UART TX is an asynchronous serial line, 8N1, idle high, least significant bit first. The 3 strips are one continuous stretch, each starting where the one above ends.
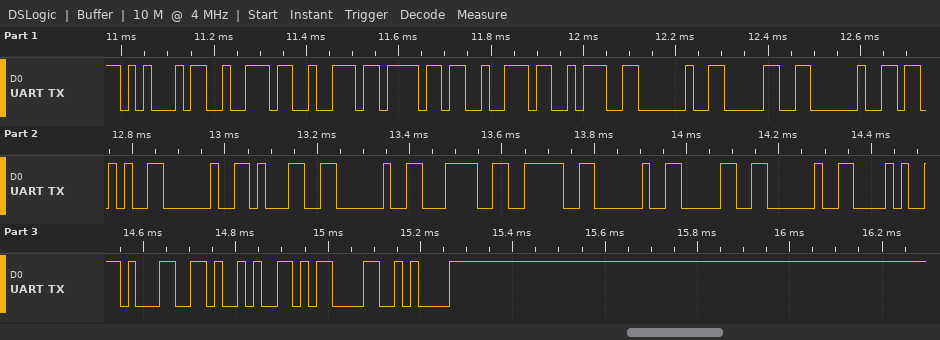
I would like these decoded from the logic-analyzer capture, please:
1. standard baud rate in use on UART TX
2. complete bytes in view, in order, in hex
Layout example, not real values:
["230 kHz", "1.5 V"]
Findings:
["57600 baud", "45 72 72 6F 72 3A 20 30 20 2B 20 31 20 3C 3E 20 30 20 28 31 29 0D 0A"]
